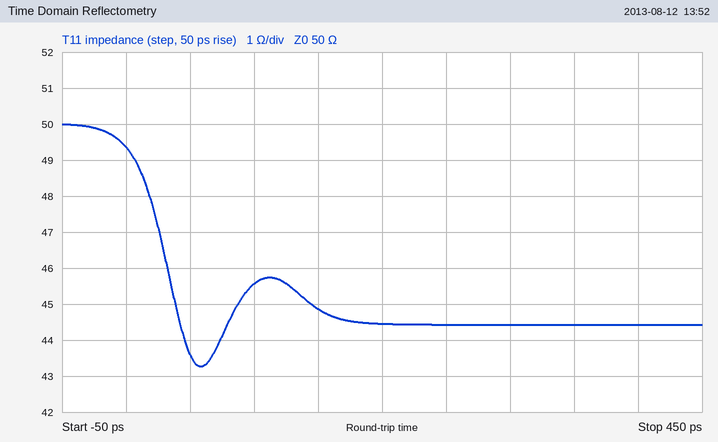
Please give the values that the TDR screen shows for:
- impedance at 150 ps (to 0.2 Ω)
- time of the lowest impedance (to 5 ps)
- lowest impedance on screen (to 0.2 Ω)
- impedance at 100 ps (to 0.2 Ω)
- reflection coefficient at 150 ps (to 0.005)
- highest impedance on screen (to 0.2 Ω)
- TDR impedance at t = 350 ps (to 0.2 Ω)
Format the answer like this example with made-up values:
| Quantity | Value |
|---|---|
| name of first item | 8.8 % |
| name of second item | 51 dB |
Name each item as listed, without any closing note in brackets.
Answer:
| Quantity | Value |
|---|---|
| impedance at 150 ps | 44.8 Ω |
| time of the lowest impedance | 60 ps |
| lowest impedance on screen | 43.2 Ω |
| impedance at 100 ps | 45.6 Ω |
| reflection coefficient at 150 ps | -0.055 |
| highest impedance on screen | 50.0 Ω |
| TDR impedance at t = 350 ps | 44.4 Ω |
